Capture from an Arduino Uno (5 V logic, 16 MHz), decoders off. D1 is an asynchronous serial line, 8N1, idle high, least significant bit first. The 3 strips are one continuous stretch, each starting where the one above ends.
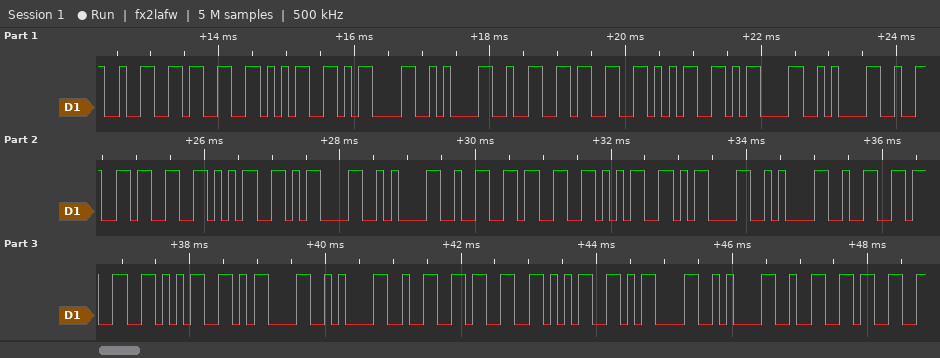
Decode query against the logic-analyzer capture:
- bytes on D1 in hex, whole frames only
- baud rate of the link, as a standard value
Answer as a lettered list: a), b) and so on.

a) 32 33 35 0D 0A 32 33 35 0D 0A 32 33 35 0D 0A 32 33 35 0D 0A 32 33 35 0D 0A 32 33 35 0D 0A 32 33
b) 9600 baud
